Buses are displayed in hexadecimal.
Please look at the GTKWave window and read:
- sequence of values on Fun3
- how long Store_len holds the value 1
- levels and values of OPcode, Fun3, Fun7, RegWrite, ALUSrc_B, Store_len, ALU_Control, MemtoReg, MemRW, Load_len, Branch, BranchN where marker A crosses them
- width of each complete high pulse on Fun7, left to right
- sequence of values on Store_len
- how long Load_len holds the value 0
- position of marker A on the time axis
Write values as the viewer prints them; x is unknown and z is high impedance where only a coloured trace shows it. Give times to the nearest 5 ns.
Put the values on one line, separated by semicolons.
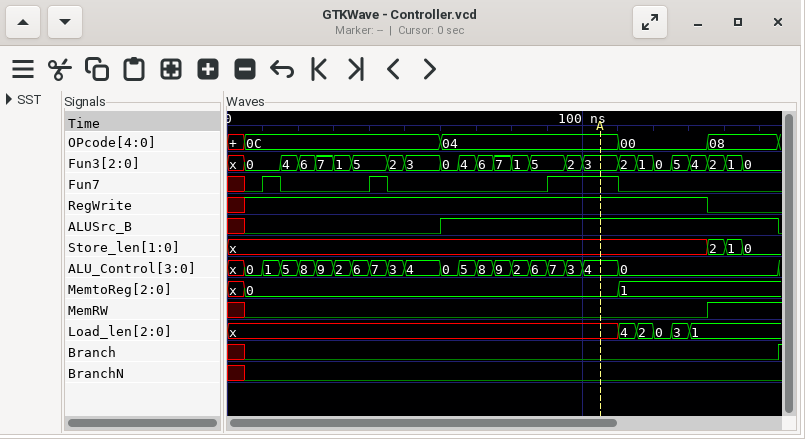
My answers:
x, 0, 4, 6, 7, 1, 5, 2, 3, 0, 4, 6, 7, 1, 5, 2, 3, 2, 1, 0, 5, 4, 2, 1, 0; 5 ns; OPcode=04, Fun3=3, Fun7=1, RegWrite=1, ALUSrc_B=1, Store_len=x, ALU_Control=4, MemtoReg=0, MemRW=0, Load_len=x, Branch=0, BranchN=0; 5 ns, 5 ns, 20 ns; x, 2, 1, 0; 5 ns; 105 ns
